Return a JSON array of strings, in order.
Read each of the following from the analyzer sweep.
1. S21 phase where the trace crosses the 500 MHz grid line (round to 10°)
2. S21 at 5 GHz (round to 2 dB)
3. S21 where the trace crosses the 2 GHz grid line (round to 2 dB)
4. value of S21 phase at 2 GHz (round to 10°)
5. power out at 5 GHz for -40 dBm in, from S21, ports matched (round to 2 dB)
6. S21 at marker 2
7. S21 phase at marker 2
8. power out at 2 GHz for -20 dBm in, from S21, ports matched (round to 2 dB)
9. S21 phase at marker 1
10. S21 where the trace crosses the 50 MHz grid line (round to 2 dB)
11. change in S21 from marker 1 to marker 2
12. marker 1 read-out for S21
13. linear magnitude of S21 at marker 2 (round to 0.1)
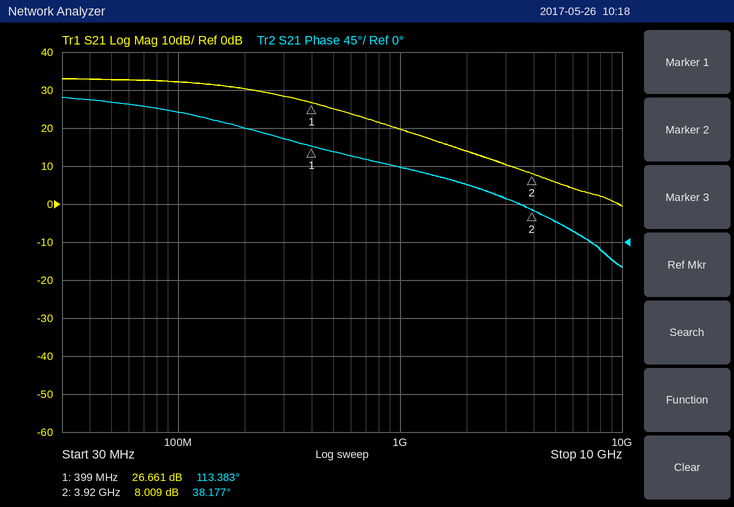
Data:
["110°", "6 dB", "14 dB", "70°", "-34 dBm", "8.009 dB", "38.177°", "-6 dBm", "113.383°", "32 dB", "-18.652 dB", "26.661 dB", "2.5"]
